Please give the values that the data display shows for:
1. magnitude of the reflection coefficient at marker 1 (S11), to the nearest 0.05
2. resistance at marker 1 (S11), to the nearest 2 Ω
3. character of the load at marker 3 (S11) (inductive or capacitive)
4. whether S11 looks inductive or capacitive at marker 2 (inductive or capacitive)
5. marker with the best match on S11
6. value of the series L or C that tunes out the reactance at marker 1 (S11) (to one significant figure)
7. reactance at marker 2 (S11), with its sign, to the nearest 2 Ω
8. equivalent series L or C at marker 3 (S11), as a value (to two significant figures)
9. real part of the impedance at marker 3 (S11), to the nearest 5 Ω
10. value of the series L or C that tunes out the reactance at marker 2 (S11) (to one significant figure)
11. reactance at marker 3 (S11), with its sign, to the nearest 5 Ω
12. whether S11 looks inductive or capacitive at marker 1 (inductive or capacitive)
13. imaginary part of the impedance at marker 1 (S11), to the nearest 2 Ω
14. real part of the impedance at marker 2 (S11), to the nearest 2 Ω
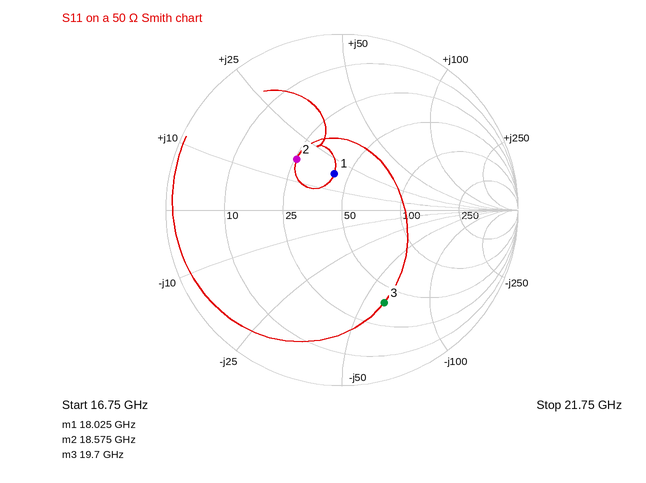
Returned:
0.20
42 Ω
capacitive
inductive
marker 1
500 fF
+18 Ω
130 fF
40 Ω
500 fF
-60 Ω
inductive
+18 Ω
26 Ω
